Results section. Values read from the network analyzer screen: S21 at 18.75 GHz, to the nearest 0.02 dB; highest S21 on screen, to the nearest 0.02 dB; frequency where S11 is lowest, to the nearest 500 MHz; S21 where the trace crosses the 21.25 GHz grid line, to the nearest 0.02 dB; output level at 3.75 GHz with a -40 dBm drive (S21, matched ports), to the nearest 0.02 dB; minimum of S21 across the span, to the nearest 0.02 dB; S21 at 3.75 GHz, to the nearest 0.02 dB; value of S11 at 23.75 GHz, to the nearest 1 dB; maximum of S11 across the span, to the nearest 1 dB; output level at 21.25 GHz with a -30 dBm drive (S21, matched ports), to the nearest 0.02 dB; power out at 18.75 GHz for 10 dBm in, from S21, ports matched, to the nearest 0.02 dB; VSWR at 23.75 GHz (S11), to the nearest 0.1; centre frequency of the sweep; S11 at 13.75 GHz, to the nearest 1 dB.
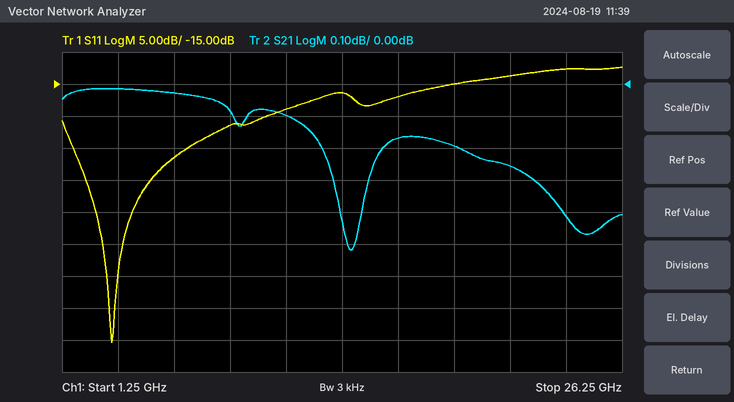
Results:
-0.20 dB
-0.02 dB
3.5 GHz
-0.26 dB
-40.02 dBm
-0.52 dB
-0.02 dB
-13 dB
-12 dB
-30.26 dBm
9.80 dBm
1.6
13.75 GHz
-16 dB
